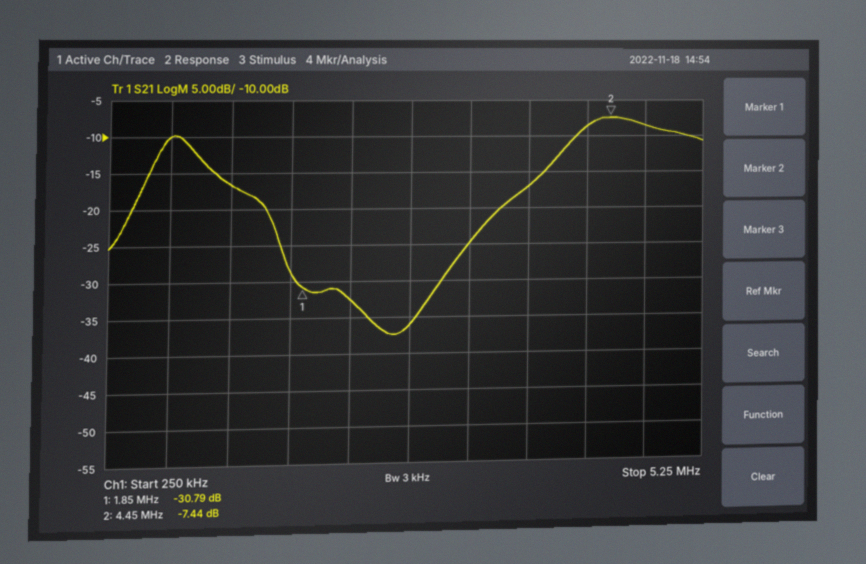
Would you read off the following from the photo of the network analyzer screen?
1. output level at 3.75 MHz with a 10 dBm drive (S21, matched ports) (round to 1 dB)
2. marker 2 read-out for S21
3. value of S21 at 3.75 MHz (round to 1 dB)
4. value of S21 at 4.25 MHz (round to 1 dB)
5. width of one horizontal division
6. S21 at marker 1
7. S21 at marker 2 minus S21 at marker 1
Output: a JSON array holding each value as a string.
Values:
["-7 dBm", "-7.44 dB", "-17 dB", "-9 dB", "500 kHz", "-30.79 dB", "23.35 dB"]
